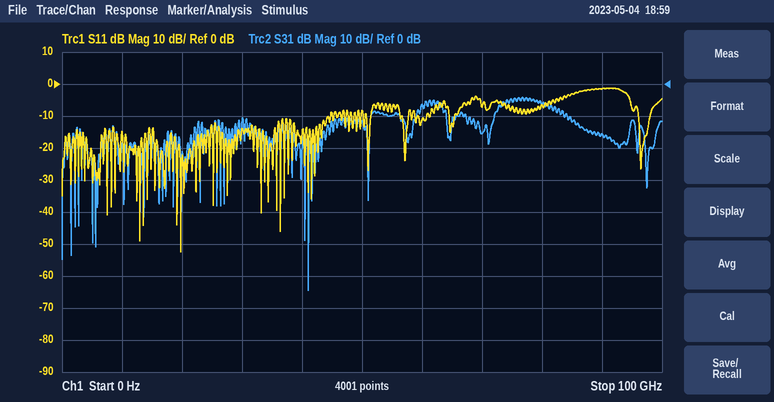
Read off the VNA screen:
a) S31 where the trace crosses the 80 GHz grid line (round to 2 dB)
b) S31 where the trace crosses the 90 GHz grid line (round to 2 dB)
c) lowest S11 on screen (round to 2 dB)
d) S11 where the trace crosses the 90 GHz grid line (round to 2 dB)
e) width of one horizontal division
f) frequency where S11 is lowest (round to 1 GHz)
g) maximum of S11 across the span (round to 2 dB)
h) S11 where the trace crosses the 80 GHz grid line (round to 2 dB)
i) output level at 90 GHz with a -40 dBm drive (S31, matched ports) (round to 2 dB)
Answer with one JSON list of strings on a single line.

["-6 dB", "-16 dB", "-52 dB", "-2 dB", "10 GHz", "20 GHz", "-2 dB", "-6 dB", "-56 dBm"]
